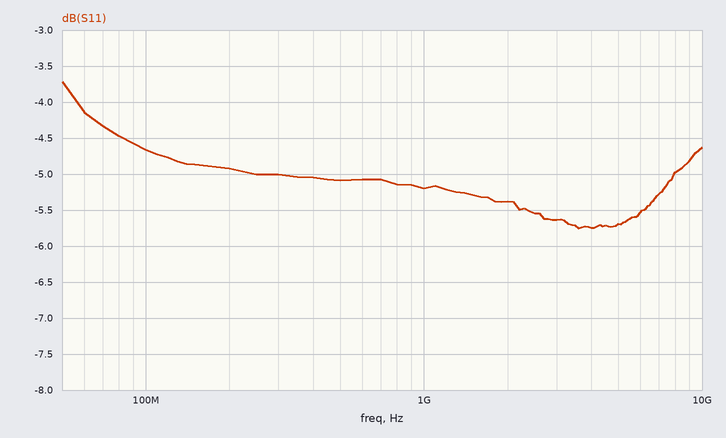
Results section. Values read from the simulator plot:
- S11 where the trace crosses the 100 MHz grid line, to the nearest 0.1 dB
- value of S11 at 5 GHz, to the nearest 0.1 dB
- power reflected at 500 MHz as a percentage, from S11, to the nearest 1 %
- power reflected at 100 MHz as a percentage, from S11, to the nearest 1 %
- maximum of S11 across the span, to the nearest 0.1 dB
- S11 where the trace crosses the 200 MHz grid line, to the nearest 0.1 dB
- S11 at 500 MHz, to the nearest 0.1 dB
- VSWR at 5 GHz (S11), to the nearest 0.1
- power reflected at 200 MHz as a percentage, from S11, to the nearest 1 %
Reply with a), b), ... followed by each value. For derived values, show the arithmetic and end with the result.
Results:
a) -4.7 dB
b) -5.7 dB
c) 10^(-5.1/10) ≈ 31 %
d) 10^(-4.7/10) ≈ 34 %
e) -3.7 dB
f) -4.9 dB
g) -5.1 dB
h) |Γ| = 10^(-5.7/20) = 0.5188; VSWR = (1 + 0.5188)/(1 − 0.5188) ≈ 3.2
i) 10^(-4.9/10) ≈ 32 %
